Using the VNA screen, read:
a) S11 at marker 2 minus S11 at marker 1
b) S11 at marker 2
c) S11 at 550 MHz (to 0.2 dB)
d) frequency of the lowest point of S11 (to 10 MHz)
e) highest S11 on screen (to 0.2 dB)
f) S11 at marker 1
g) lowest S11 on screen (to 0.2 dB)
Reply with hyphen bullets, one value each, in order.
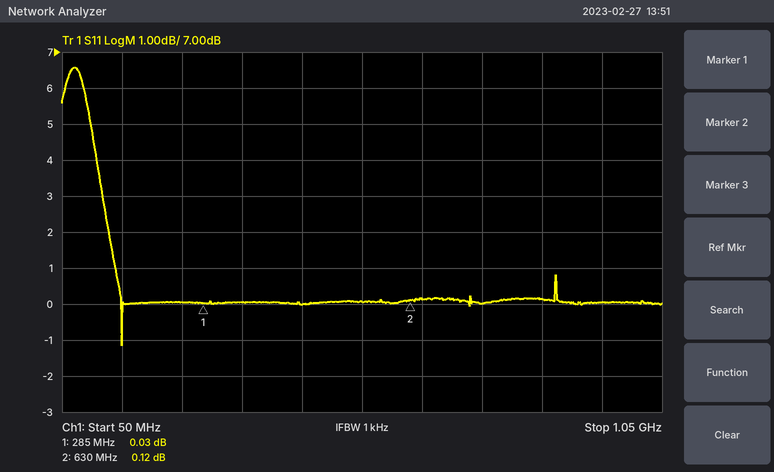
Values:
- 0.09 dB
- 0.12 dB
- 0.0 dB
- 150 MHz
- 6.6 dB
- 0.03 dB
- -1.2 dB
